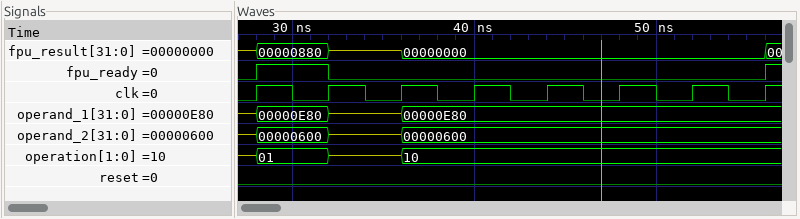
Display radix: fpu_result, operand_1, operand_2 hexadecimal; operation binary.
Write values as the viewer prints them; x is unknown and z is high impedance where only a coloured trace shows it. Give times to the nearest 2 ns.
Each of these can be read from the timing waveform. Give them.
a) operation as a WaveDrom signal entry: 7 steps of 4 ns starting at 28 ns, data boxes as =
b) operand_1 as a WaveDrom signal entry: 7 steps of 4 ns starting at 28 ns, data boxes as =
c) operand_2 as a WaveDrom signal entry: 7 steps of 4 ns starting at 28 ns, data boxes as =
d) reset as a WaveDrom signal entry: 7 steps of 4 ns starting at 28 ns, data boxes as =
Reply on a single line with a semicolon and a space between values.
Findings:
{name: 'operation', wave: '=z=....', data: '01 10'}; {name: 'operand_1', wave: '=z=....', data: '00000E80 00000E80'}; {name: 'operand_2', wave: '=z=....', data: '00000600 00000600'}; {name: 'reset', wave: '0......'}
